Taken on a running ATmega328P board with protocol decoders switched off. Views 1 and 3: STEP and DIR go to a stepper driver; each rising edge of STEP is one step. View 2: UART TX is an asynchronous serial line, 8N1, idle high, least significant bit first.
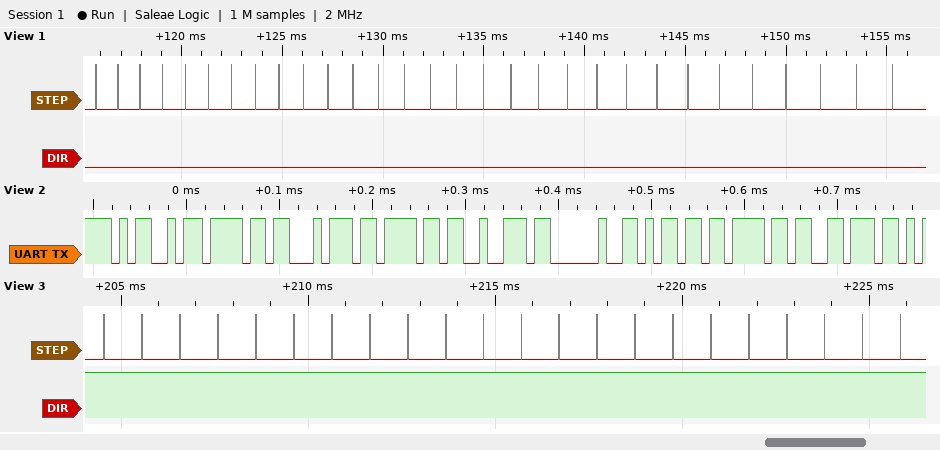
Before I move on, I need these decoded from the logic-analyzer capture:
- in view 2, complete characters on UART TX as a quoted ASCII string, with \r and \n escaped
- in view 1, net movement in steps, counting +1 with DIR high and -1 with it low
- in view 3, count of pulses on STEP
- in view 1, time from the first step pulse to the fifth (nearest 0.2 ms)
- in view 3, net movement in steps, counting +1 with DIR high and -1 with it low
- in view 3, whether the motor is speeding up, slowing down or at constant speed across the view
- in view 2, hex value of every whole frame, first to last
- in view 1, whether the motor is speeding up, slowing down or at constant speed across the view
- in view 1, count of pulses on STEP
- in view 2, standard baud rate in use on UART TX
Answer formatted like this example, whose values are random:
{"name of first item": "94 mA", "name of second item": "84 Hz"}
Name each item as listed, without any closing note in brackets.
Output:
{"in view 2, complete characters on UART TX as a quoted ASCII string, with \\r and \\n escaped": "\"Motor mov\"", "in view 1, net movement in steps, counting +1 with DIR high and -1 with it low": "-30", "in view 3, count of pulses on STEP": "22", "in view 1, time from the first step pulse to the fifth": "4.4 ms", "in view 3, net movement in steps, counting +1 with DIR high and -1 with it low": "+22", "in view 3, whether the motor is speeding up, slowing down or at constant speed across the view": "constant speed", "in view 2, hex value of every whole frame, first to last": "4D 6F 74 6F 72 20 6D 6F 76", "in view 1, whether the motor is speeding up, slowing down or at constant speed across the view": "slowing down", "in view 1, count of pulses on STEP": "30", "in view 2, standard baud rate in use on UART TX": "115200 baud"}
